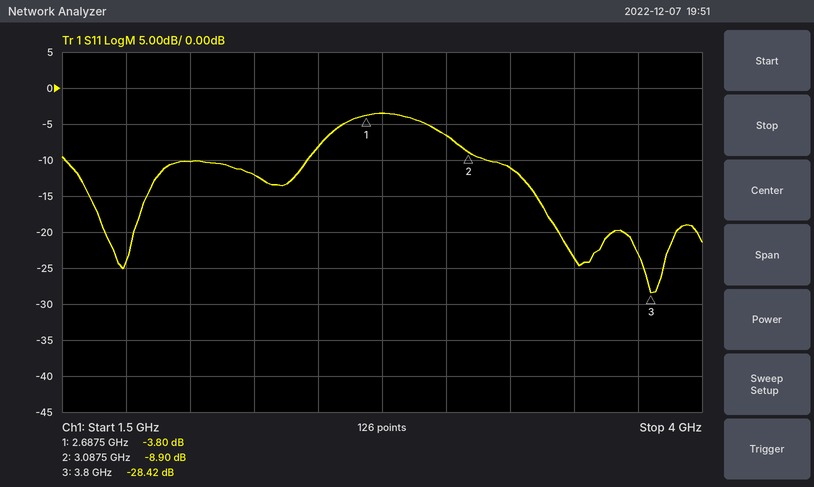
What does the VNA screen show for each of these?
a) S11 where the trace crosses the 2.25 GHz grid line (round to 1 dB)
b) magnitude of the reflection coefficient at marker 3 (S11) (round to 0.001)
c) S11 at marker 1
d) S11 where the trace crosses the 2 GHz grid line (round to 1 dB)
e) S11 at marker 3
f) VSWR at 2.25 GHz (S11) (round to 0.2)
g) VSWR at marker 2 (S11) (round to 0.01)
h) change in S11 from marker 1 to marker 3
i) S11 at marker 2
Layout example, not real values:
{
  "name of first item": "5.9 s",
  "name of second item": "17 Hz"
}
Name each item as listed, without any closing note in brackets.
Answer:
{
  "S11 where the trace crosses the 2.25 GHz grid line": "-12 dB",
  "magnitude of the reflection coefficient at marker 3 (S11)": "0.038",
  "S11 at marker 1": "-3.80 dB",
  "S11 where the trace crosses the 2 GHz grid line": "-10 dB",
  "S11 at marker 3": "-28.42 dB",
  "VSWR at 2.25 GHz (S11)": "1.6",
  "VSWR at marker 2 (S11)": "2.12",
  "change in S11 from marker 1 to marker 3": "-24.62 dB",
  "S11 at marker 2": "-8.90 dB"
}
